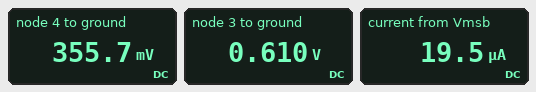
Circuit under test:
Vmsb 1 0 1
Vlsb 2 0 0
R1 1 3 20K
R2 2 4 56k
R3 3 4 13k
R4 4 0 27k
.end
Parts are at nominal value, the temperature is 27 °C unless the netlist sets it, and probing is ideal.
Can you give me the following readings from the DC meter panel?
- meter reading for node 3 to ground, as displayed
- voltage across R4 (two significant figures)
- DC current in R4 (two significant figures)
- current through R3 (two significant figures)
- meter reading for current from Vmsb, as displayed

0.610 V
360 mV
13 µA
20 µA
19.5 µA
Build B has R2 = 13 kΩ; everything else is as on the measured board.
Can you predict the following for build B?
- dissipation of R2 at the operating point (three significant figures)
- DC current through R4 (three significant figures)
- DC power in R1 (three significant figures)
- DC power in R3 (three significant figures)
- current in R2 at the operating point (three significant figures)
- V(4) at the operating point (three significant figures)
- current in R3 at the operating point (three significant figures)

3.39 µW
7.78 µA
11.5 µW
7.45 µW
16.2 µA
210 mV
23.9 µA
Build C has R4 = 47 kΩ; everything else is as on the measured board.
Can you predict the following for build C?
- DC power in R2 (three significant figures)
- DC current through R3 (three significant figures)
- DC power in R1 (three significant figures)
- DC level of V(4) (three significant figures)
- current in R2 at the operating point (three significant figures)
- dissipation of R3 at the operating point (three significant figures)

3.40 µW
17.1 µA
5.83 µW
436 mV
7.79 µA
3.79 µW
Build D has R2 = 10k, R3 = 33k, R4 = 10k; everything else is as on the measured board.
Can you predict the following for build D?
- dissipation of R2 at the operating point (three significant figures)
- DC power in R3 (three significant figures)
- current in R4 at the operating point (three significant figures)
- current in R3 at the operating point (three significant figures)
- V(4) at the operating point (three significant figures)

743 nW
9.81 µW
8.62 µA
17.2 µA
86.2 mV
